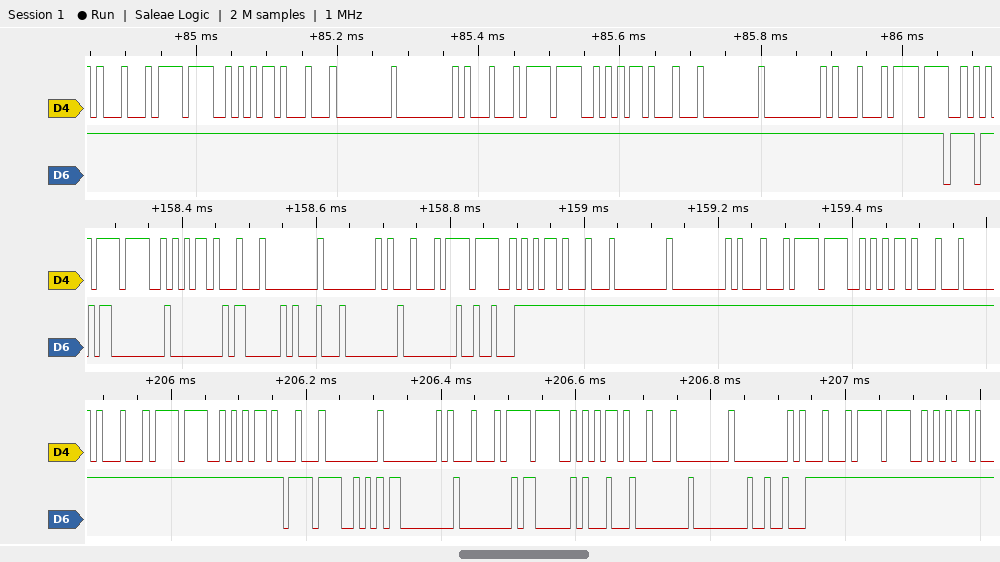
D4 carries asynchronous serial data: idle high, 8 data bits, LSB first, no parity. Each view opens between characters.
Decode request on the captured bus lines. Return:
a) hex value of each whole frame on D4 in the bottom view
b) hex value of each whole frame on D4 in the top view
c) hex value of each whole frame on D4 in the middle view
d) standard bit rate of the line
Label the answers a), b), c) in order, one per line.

a) 11, EF, AA, 11, 00, 00, 11, EF, AA, 11, 00, 00, 11, EF, AA
b) 11, EF, AA, 11, 00, 00, 11, EF, AA, 11, 00, 00, 11, EF
c) EF, AA, 11, 00, 00, 11, EF, AA, 11, 00, 00, 11, EF, AA, 11
d) 115200 baud
